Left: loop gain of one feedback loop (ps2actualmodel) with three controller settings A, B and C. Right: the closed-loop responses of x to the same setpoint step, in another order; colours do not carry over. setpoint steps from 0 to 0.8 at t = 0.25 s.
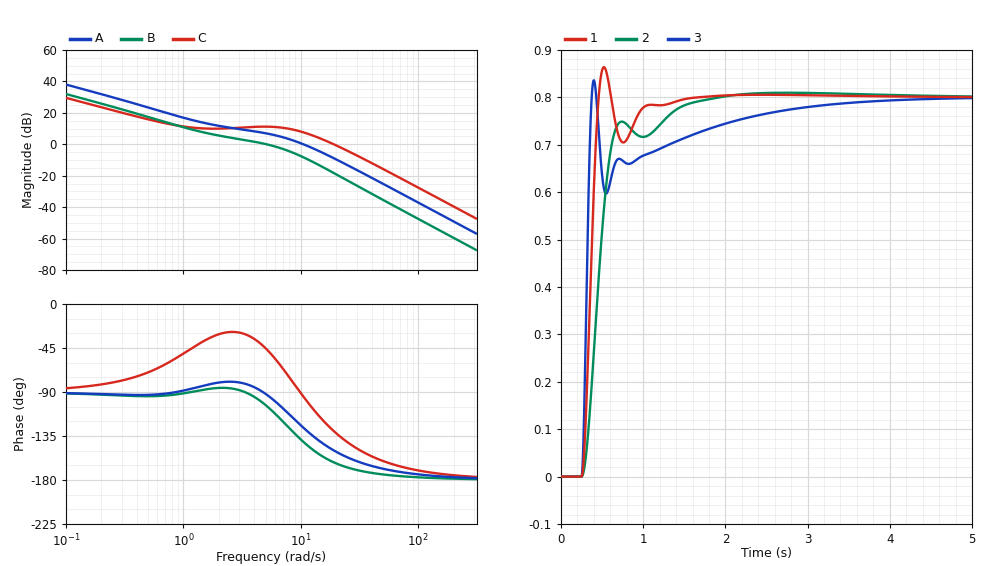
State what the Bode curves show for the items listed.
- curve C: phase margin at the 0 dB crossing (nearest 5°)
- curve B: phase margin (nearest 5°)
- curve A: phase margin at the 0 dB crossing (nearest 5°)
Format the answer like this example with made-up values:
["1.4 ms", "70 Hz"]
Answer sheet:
["50°", "75°", "55°"]
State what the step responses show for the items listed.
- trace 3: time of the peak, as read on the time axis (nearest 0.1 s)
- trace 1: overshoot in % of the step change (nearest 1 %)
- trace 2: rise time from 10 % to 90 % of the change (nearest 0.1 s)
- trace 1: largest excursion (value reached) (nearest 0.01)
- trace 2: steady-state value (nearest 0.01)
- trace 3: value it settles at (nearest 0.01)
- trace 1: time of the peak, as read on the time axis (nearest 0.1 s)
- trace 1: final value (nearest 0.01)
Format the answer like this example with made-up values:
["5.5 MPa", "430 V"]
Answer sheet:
["0.4 s", "8 %", "0.3 s", "0.86", "0.80", "0.80", "0.5 s", "0.80"]
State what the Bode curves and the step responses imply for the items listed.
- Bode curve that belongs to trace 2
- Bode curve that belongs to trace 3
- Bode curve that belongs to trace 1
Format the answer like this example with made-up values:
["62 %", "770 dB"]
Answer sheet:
["B", "C", "A"]
